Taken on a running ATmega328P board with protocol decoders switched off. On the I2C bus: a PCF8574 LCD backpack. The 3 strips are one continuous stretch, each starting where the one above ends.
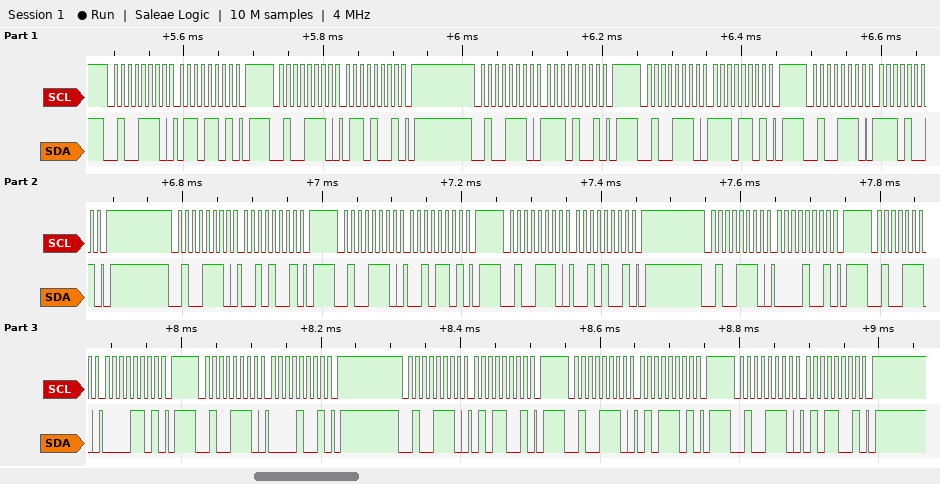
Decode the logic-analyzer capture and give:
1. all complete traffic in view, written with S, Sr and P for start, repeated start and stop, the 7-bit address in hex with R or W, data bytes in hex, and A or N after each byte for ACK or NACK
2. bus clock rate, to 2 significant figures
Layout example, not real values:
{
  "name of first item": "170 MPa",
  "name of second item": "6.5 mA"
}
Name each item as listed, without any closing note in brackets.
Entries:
{
  "all complete traffic in view, written with S, Sr and P for start, repeated start and stop, the 7-bit address in hex with R or W, data bytes in hex, and A or N after each byte for ACK or NACK": "S 27W A 6D A P S 27W A 69 A P S 27W A E9 A P S 27W A ED A P S 27W A E9 A P S 27W A 29 A P S 27W A 2D A P S 27W A 29 A P S 27W A 09 A P S 27W A 0D A P S 27W A 09 A P S 27W A 59 A P S 27W A 5D A P S 27W A 59 A P",
  "bus clock rate, to 2 significant figures": "100 kHz"
}
